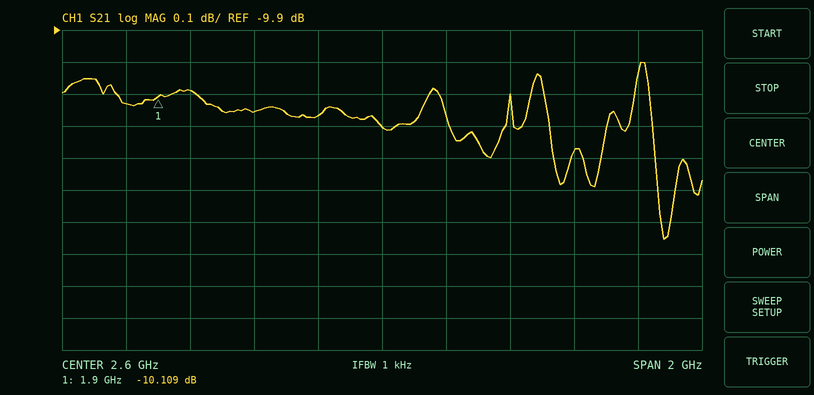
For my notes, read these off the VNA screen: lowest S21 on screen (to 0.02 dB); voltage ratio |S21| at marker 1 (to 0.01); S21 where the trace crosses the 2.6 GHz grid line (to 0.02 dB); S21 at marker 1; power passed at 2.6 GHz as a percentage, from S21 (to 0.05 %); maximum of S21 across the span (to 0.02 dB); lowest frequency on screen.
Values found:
-10.56 dB
0.31
-10.20 dB
-10.109 dB
9.55 %
-10.00 dB
1.6 GHz
